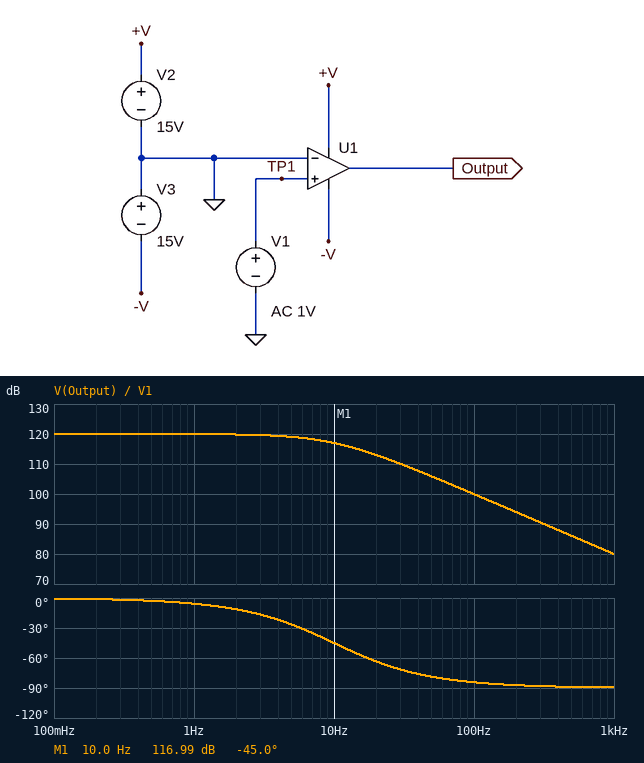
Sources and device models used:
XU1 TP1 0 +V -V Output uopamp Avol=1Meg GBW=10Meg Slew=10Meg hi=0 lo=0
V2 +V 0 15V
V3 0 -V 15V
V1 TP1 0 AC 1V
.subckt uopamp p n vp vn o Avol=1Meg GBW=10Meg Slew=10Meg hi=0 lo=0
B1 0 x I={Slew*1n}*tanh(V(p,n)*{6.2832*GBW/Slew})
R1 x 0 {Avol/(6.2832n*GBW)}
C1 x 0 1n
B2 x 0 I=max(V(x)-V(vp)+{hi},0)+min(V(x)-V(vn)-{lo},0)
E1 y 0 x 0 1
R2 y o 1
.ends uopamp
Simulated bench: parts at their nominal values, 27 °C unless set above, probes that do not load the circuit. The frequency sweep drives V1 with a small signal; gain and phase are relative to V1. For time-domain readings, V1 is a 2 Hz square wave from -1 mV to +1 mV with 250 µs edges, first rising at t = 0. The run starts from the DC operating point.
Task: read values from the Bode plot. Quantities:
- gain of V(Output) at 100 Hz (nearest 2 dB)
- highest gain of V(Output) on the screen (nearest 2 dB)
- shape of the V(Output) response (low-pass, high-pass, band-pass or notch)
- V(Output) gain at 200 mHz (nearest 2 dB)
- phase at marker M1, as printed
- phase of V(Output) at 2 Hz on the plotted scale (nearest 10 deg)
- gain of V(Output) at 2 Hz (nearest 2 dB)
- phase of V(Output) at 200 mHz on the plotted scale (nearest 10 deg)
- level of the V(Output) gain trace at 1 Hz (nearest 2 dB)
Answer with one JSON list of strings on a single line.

["100 dB", "120 dB", "low-pass", "120 dB", "-45.0 deg", "-10 deg", "120 dB", "0 deg", "120 dB"]
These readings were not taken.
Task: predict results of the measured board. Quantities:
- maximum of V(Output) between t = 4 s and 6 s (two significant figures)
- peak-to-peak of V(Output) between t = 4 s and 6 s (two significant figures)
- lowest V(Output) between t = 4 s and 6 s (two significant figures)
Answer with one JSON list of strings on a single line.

["15 V", "30 V", "-15 V"]
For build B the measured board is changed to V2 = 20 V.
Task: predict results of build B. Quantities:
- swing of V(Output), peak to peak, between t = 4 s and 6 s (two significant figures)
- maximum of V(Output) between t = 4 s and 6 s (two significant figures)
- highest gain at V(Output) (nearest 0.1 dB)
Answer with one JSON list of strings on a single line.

["35 V", "20 V", "120.0 dB"]
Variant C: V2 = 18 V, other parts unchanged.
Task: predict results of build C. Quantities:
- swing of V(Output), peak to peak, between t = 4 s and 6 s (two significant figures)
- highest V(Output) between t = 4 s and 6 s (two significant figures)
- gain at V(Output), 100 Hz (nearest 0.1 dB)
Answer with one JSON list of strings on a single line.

["33 V", "18 V", "100.0 dB"]
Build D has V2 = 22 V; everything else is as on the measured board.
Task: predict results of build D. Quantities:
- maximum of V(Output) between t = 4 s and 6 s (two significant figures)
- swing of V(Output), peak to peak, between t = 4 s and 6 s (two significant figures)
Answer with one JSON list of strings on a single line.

["22 V", "37 V"]
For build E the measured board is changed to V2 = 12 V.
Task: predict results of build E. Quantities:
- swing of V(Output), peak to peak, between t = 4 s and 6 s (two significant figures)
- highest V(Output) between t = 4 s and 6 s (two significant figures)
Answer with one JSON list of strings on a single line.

["27 V", "12 V"]
